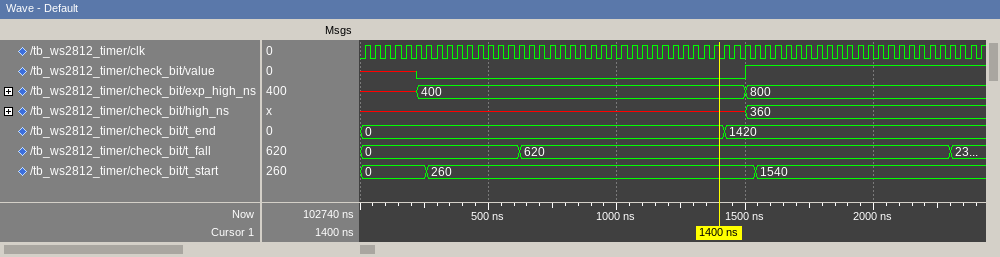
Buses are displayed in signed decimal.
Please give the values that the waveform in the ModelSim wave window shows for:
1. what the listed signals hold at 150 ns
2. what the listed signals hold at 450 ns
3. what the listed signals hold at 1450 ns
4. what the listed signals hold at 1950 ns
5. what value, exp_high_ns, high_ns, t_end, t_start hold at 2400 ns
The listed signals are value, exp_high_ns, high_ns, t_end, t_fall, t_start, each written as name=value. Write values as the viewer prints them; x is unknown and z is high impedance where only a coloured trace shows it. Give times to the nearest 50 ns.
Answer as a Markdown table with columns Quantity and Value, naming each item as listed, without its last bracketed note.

| Quantity | Value |
|---|---|
| what the listed signals hold at 150 ns | value=x, exp_high_ns=x, high_ns=x, t_end=0, t_fall=0, t_start=0 |
| what the listed signals hold at 450 ns | value=0, exp_high_ns=400, high_ns=x, t_end=0, t_fall=0, t_start=260 |
| what the listed signals hold at 1450 ns | value=0, exp_high_ns=400, high_ns=x, t_end=1420, t_fall=620, t_start=260 |
| what the listed signals hold at 1950 ns | value=1, exp_high_ns=800, high_ns=360, t_end=1420, t_fall=620, t_start=1540 |
| what value, exp_high_ns, high_ns, t_end, t_start hold at 2400 ns | value=1, exp_high_ns=800, high_ns=360, t_end=1420, t_start=1540 |
